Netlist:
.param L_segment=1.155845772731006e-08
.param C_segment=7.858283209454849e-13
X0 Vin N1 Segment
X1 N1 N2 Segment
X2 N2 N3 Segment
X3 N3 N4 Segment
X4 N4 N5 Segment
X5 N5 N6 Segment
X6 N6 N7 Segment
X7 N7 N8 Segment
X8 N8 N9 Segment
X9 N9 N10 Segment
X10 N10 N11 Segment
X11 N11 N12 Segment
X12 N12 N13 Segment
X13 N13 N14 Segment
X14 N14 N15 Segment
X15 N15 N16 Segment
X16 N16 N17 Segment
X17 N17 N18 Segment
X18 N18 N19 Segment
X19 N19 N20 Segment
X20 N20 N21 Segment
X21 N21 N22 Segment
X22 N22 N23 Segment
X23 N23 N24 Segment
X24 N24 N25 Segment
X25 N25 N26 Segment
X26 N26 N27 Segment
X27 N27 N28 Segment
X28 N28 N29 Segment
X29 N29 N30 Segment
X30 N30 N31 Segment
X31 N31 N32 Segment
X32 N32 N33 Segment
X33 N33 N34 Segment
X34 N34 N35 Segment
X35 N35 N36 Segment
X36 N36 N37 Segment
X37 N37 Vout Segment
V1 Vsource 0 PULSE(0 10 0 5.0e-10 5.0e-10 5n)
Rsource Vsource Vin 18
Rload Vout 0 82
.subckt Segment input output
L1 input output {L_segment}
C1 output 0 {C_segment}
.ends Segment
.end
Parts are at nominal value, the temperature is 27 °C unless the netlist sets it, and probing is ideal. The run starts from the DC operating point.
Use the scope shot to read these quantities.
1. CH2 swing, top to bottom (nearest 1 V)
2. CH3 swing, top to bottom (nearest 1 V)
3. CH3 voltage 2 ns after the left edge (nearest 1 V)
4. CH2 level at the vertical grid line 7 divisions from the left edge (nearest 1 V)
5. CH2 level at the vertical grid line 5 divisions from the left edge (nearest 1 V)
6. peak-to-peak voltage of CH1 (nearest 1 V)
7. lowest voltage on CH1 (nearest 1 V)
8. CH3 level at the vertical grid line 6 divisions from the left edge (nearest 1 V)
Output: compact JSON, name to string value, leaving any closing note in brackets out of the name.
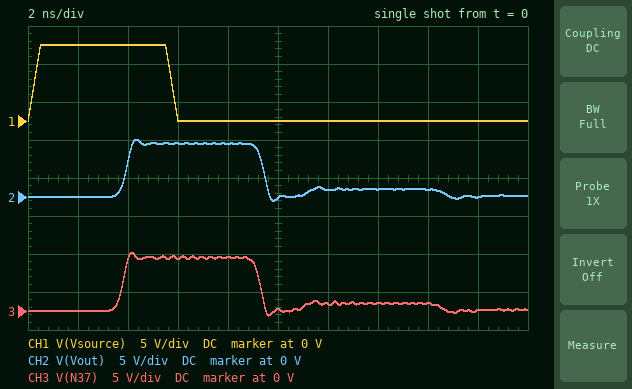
{"CH2 swing, top to bottom": "8 V", "CH3 swing, top to bottom": "8 V", "CH3 voltage 2 ns after the left edge": "0 V", "CH2 level at the vertical grid line 7 divisions from the left edge": "1 V", "CH2 level at the vertical grid line 5 divisions from the left edge": "0 V", "peak-to-peak voltage of CH1": "10 V", "lowest voltage on CH1": "0 V", "CH3 level at the vertical grid line 6 divisions from the left edge": "1 V"}
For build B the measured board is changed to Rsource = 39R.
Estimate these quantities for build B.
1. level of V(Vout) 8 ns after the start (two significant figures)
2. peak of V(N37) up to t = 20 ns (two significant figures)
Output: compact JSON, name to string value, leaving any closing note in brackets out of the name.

{"level of V(Vout) 8 ns after the start": "6.1 V", "peak of V(N37) up to t = 20 ns": "6.6 V"}
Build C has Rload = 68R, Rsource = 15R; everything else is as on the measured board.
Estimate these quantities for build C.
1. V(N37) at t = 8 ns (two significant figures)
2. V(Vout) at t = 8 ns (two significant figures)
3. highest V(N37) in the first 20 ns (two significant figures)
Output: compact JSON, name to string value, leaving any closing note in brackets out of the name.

{"V(N37) at t = 8 ns": "6.5 V", "V(Vout) at t = 8 ns": "6.4 V", "highest V(N37) in the first 20 ns": "7.2 V"}
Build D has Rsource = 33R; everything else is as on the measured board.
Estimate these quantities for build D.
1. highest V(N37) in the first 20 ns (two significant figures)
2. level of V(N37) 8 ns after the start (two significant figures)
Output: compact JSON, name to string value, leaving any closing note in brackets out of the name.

{"highest V(N37) in the first 20 ns": "6.9 V", "level of V(N37) 8 ns after the start": "6.4 V"}
